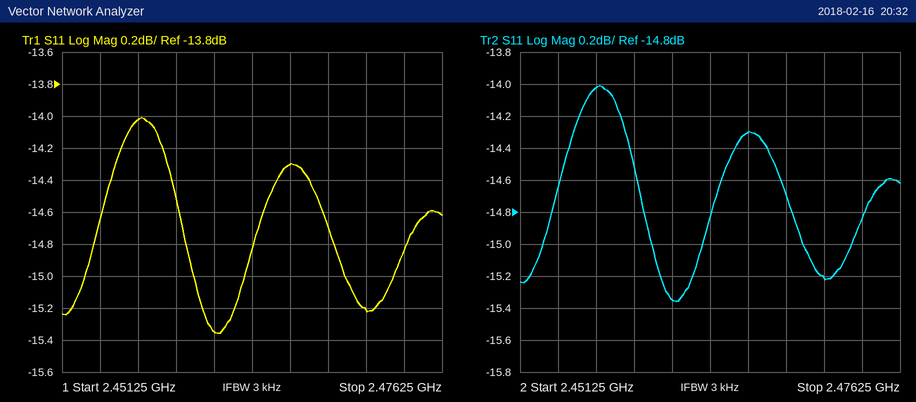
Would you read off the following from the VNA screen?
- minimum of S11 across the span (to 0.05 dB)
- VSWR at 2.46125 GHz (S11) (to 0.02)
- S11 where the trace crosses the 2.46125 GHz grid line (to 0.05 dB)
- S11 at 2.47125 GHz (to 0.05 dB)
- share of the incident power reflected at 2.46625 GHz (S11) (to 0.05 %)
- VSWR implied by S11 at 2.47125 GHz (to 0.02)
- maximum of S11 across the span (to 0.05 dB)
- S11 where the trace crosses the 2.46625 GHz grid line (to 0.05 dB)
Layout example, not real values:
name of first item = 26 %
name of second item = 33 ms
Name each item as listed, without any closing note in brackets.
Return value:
minimum of S11 across the span = -15.35 dB
VSWR at 2.46125 GHz (S11) = 1.42
S11 where the trace crosses the 2.46125 GHz grid line = -15.35 dB
S11 at 2.47125 GHz = -15.20 dB
share of the incident power reflected at 2.46625 GHz (S11) = 3.70 %
VSWR implied by S11 at 2.47125 GHz = 1.42
maximum of S11 across the span = -14.00 dB
S11 where the trace crosses the 2.46625 GHz grid line = -14.30 dB
